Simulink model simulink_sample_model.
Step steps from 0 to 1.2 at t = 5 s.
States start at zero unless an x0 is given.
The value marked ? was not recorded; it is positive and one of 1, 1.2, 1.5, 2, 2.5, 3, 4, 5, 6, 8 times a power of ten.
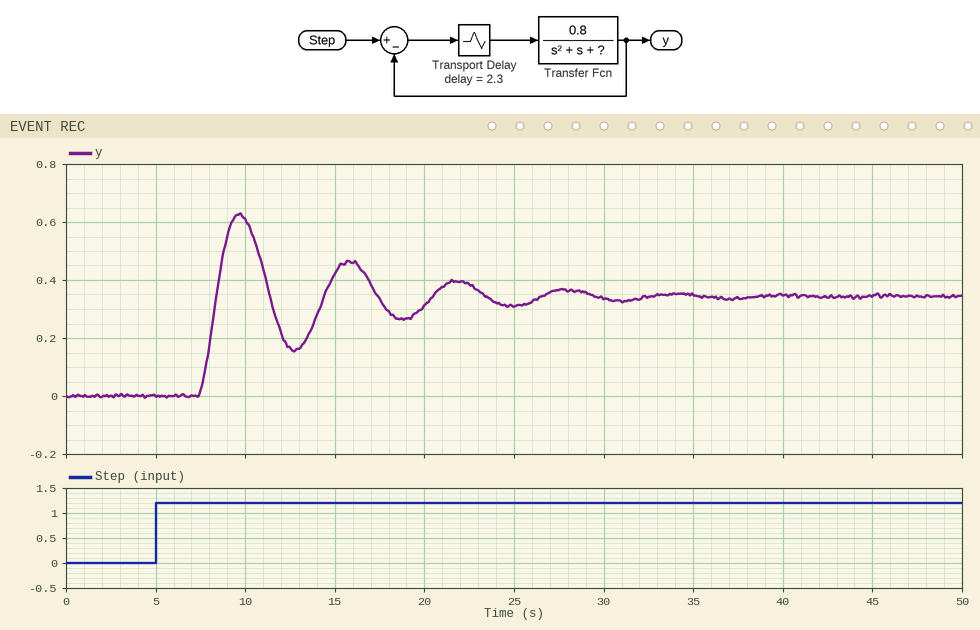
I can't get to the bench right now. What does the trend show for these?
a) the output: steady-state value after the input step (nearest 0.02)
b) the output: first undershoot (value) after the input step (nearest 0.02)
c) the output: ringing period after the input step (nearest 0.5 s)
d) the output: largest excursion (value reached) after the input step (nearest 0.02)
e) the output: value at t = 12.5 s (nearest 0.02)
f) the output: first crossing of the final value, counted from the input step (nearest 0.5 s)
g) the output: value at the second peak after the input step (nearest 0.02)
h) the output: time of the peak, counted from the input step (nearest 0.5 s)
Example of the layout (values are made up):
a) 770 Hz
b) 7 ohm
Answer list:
a) 0.34
b) 0.16
c) 6.0 s
d) 0.62
e) 0.16
f) 3.5 s
g) 0.46
h) 4.5 s
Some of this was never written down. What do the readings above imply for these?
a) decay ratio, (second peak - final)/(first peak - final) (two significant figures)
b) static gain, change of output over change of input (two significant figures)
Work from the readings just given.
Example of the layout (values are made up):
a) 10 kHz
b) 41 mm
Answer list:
a) 0.43
b) 0.28
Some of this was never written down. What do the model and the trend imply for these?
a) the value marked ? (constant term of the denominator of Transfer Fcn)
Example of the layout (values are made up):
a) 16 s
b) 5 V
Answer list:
a) 2
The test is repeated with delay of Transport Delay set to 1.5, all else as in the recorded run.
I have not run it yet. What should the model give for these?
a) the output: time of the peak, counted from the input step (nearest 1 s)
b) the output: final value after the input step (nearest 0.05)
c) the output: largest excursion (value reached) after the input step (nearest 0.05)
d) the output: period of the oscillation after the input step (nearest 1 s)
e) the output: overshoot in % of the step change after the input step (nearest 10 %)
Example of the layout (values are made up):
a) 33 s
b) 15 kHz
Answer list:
a) 4 s
b) 0.35
c) 0.60
d) 5 s
e) 80 %
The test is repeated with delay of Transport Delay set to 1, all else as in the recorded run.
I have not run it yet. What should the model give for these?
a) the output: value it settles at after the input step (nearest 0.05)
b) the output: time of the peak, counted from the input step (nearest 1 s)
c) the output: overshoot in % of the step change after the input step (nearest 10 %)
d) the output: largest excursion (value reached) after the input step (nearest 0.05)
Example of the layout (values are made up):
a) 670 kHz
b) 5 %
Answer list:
a) 0.35
b) 3 s
c) 70 %
d) 0.60
